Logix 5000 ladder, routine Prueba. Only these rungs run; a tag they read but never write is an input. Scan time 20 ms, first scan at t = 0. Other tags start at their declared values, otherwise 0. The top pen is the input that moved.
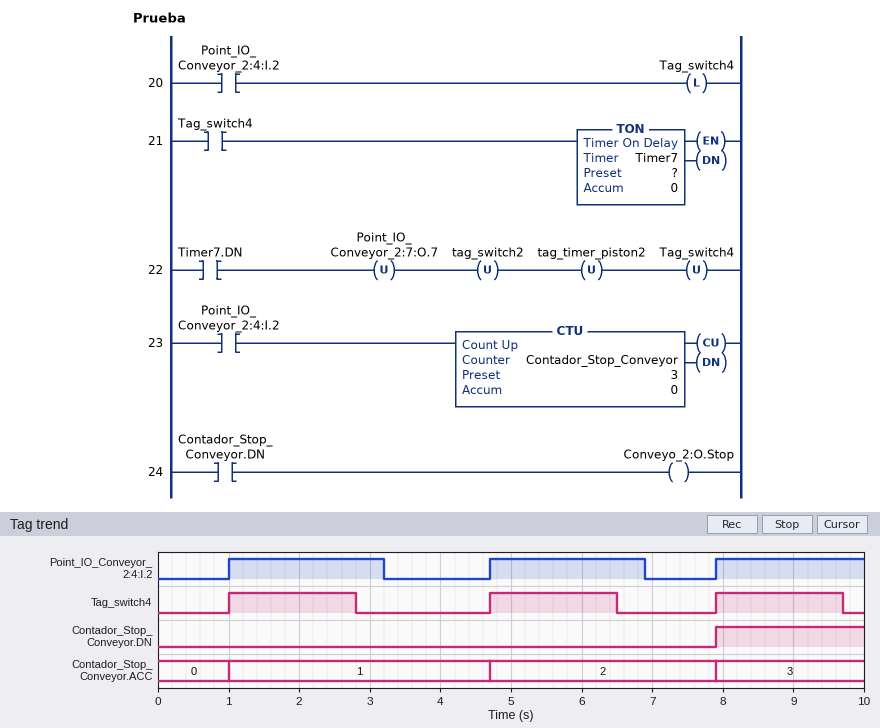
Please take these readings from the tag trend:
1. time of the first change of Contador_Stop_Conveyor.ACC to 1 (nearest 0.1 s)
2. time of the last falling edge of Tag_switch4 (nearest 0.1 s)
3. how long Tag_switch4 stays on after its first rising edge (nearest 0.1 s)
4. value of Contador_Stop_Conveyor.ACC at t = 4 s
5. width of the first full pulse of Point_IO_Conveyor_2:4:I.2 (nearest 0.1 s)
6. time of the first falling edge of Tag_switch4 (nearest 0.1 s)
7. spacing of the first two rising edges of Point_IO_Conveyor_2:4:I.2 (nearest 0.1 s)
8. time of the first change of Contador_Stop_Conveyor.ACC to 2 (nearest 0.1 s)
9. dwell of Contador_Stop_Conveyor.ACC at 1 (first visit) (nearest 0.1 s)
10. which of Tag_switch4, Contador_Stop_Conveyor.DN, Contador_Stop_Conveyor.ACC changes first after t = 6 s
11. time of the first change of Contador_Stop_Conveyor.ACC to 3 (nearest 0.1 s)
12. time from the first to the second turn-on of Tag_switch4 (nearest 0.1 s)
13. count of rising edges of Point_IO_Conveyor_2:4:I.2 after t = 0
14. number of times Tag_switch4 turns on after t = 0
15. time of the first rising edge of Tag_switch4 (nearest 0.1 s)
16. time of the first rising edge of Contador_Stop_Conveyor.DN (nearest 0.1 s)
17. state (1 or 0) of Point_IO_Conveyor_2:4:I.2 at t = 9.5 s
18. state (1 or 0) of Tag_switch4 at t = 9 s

1.0 s
9.7 s
1.8 s
1
2.2 s
2.8 s
3.7 s
4.7 s
3.7 s
Tag_switch4
7.9 s
3.7 s
3
3
1.0 s
7.9 s
1
1
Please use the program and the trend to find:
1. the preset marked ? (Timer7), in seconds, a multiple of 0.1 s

1.8 s
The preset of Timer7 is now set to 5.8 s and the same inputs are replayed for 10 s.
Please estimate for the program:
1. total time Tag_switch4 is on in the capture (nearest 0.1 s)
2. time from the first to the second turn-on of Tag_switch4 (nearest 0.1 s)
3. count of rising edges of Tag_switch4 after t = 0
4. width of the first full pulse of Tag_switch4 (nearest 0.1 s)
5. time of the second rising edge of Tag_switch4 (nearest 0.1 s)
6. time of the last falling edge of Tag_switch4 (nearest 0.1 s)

7.9 s
6.9 s
2
5.8 s
7.9 s
6.8 s
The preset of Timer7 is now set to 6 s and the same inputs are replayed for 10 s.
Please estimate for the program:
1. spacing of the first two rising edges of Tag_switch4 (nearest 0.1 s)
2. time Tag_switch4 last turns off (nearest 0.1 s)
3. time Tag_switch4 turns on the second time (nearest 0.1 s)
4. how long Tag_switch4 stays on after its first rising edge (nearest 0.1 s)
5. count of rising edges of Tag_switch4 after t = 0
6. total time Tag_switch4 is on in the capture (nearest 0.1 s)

6.9 s
7.0 s
7.9 s
6.0 s
2
8.1 s
